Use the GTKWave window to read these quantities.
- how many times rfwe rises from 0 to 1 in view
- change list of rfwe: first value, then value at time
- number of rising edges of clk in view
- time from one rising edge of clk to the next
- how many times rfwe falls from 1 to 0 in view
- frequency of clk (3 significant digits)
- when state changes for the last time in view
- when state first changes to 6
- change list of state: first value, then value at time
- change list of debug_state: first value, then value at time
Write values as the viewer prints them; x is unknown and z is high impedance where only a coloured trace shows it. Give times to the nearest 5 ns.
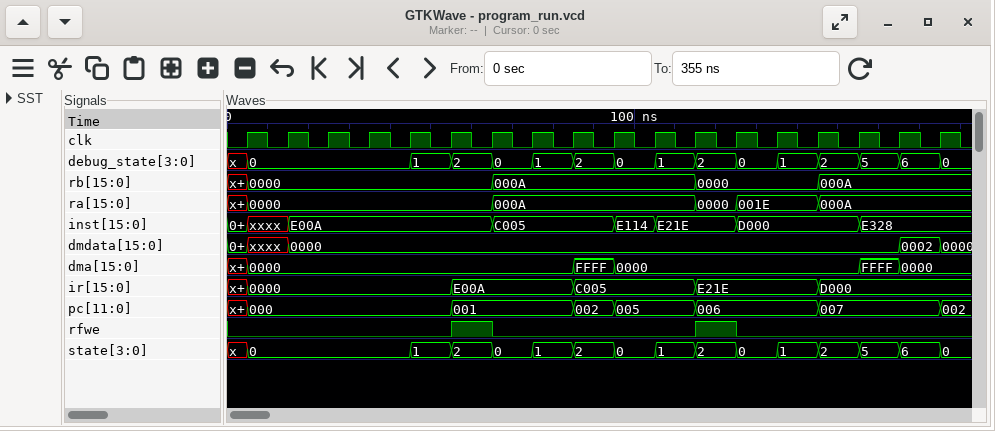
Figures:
2
0, 1 at 55 ns, 0 at 65 ns, 1 at 115 ns, 0 at 125 ns
18
10 ns
2
100 MHz
175 ns
165 ns
x, 0 at 5 ns, 1 at 45 ns, 2 at 55 ns, 0 at 65 ns, 1 at 75 ns, 2 at 85 ns, 0 at 95 ns, 1 at 105 ns, 2 at 115 ns, 0 at 125 ns, 1 at 135 ns, 2 at 145 ns, 5 at 155 ns, 6 at 165 ns, 0 at 175 ns
x, 0 at 5 ns, 1 at 45 ns, 2 at 55 ns, 0 at 65 ns, 1 at 75 ns, 2 at 85 ns, 0 at 95 ns, 1 at 105 ns, 2 at 115 ns, 0 at 125 ns, 1 at 135 ns, 2 at 145 ns, 5 at 155 ns, 6 at 165 ns, 0 at 175 ns
